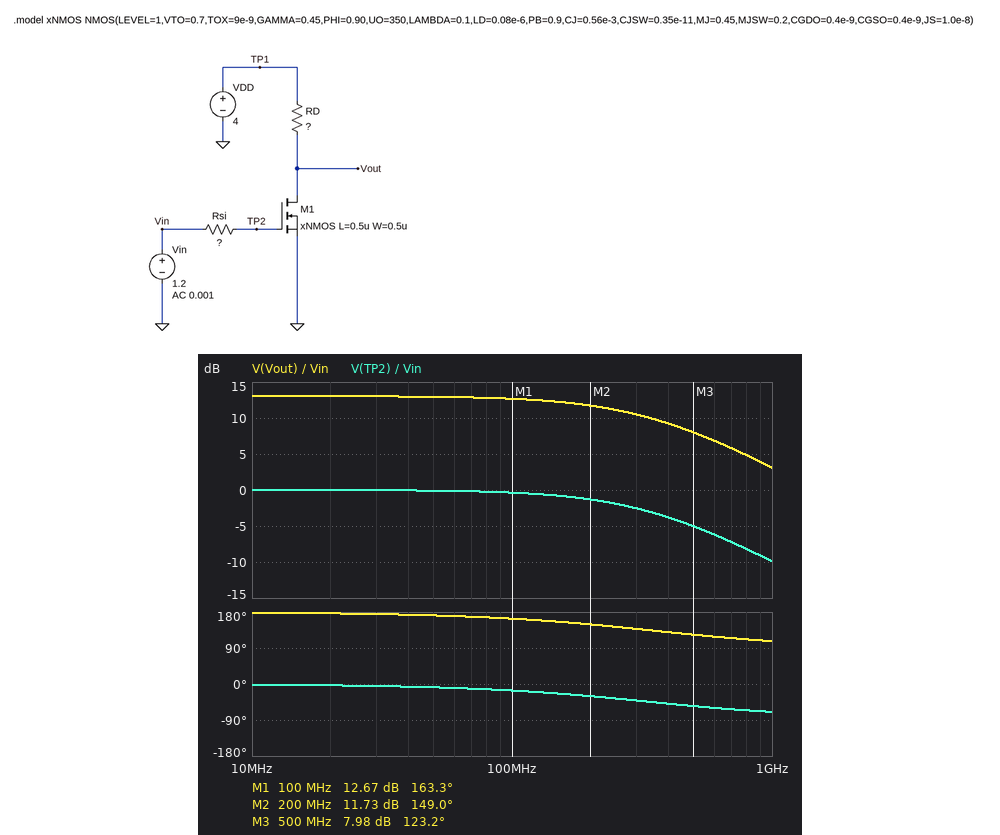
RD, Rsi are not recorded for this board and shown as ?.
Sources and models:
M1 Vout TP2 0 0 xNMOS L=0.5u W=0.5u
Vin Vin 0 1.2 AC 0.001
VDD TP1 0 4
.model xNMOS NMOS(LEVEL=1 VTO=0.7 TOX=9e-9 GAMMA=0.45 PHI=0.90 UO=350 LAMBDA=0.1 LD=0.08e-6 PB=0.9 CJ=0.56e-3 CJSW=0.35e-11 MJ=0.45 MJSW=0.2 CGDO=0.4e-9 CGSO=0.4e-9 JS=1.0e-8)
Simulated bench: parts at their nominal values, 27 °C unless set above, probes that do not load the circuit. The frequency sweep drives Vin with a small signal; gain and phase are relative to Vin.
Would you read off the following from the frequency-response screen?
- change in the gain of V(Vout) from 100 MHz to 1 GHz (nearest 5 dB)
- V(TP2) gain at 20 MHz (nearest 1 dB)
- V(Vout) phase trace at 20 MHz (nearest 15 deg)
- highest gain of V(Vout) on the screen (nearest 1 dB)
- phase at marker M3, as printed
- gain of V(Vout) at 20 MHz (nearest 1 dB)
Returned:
-10 dB
0 dB
180 deg
13 dB
123.2 deg
13 dB
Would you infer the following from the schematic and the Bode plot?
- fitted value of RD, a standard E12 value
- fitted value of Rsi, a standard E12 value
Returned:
39 kΩ
270 kΩ
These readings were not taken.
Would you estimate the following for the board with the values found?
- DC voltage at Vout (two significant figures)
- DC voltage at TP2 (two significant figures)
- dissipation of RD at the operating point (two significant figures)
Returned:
2.8 V
1.2 V
39 µW
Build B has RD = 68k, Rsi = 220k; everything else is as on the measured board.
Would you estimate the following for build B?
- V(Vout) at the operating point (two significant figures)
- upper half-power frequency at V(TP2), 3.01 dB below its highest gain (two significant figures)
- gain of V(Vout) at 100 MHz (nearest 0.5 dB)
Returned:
2.0 V
320 MHz
16.5 dB
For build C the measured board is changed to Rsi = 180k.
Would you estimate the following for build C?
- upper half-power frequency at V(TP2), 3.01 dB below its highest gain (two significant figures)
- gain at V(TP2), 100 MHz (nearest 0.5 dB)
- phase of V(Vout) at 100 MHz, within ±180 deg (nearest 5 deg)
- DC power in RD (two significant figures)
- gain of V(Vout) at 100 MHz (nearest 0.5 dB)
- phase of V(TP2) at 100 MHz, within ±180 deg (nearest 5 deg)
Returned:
500 MHz
0 dB
170 deg
39 µW
13.0 dB
-10 deg
